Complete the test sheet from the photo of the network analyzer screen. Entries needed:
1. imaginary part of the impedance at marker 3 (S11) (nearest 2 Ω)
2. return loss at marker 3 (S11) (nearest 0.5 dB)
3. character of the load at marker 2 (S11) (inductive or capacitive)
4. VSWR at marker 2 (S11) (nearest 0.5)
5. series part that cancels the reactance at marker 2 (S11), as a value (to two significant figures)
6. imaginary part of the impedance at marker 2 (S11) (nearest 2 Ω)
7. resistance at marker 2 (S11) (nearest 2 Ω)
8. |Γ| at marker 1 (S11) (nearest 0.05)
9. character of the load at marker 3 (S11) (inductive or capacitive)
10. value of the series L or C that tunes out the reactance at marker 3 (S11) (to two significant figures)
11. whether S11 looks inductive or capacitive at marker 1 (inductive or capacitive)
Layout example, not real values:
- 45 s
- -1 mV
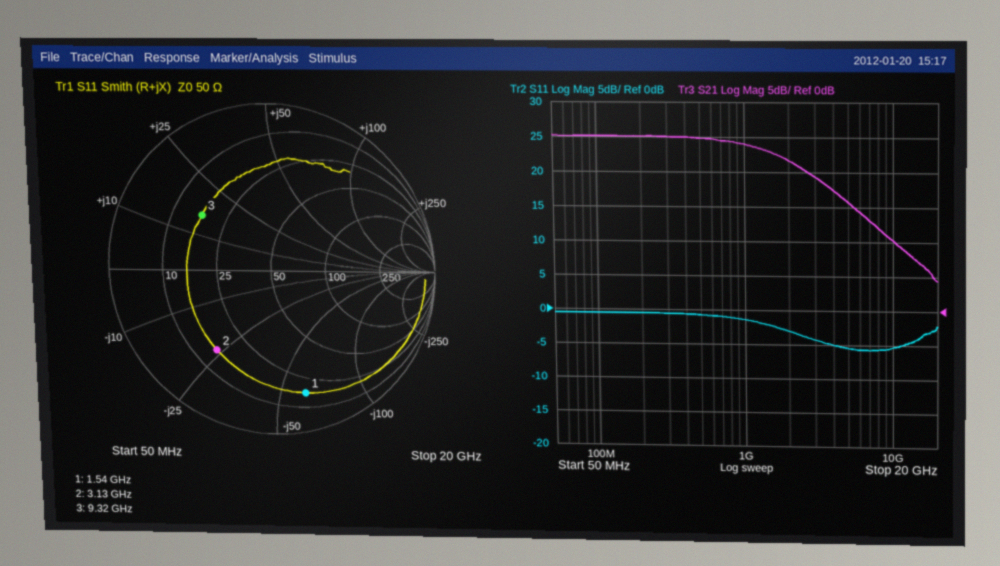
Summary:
- +16 Ω
- 5.5 dB
- capacitive
- 4.0
- 1.2 nH
- -24 Ω
- 16 Ω
- 0.75
- inductive
- 1.1 pF
- capacitive
